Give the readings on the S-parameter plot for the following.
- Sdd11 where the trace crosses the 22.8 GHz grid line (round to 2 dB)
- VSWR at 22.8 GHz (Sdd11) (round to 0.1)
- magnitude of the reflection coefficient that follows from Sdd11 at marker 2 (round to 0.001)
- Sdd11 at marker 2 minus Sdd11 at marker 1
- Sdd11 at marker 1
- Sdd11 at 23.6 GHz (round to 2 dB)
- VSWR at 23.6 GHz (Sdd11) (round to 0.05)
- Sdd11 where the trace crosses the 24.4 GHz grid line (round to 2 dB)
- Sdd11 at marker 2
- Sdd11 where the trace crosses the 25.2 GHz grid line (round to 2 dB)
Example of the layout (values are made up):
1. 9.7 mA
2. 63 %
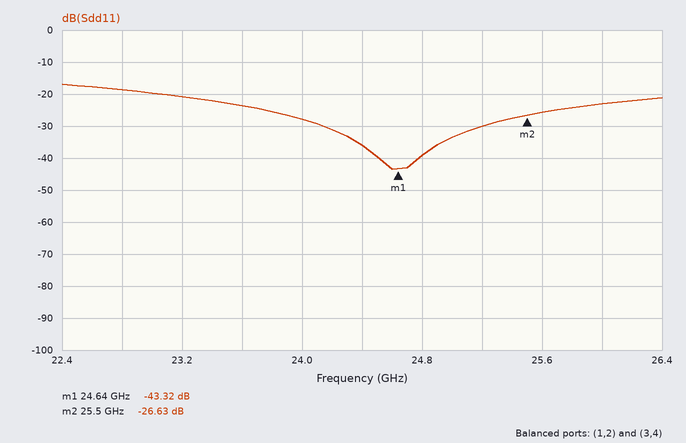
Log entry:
1. -18 dB
2. 1.3
3. 0.047
4. 16.69 dB
5. -43.32 dB
6. -24 dB
7. 1.15
8. -36 dB
9. -26.63 dB
10. -30 dB
